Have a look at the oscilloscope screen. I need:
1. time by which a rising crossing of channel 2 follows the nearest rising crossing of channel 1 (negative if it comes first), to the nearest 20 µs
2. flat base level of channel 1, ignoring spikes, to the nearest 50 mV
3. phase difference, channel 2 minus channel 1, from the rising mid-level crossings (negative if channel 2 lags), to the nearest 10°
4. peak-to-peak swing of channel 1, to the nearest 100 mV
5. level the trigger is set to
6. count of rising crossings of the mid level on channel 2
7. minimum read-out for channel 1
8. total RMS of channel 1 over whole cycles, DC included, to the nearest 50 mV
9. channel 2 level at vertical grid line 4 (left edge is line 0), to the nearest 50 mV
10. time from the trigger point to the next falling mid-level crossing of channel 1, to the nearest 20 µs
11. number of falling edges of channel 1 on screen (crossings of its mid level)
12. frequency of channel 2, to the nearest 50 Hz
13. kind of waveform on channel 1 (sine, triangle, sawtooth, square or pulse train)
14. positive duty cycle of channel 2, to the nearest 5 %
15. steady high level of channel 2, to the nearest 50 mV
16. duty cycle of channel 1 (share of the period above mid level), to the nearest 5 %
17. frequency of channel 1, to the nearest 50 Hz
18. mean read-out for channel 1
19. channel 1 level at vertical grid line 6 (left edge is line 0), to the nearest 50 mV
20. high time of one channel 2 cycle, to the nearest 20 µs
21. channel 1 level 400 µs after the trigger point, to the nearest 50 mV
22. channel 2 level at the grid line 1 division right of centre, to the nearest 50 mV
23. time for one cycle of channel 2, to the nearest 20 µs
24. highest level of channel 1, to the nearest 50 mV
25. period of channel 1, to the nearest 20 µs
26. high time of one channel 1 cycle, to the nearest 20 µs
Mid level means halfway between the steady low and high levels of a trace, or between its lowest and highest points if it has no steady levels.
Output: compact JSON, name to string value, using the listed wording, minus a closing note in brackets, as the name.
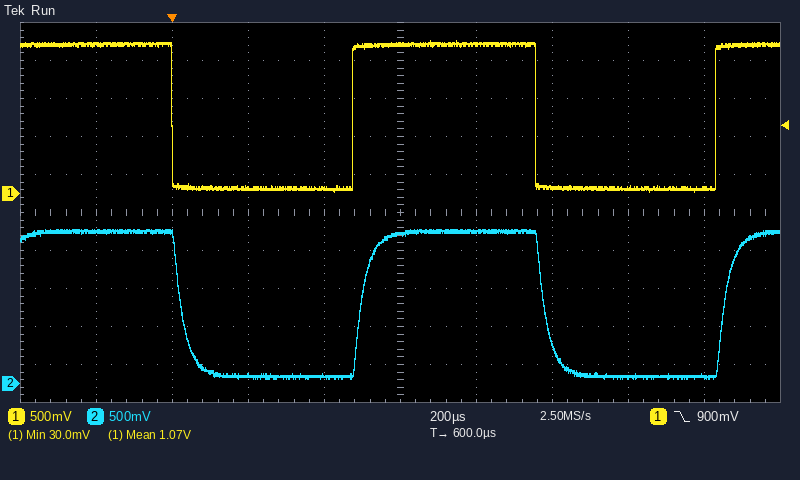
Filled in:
{"time by which a rising crossing of channel 2 follows the nearest rising crossing of channel 1 (negative if it comes first), to the nearest 20 µs": "+20 µs", "flat base level of channel 1, ignoring spikes, to the nearest 50 mV": "50 mV", "phase difference, channel 2 minus channel 1, from the rising mid-level crossings (negative if channel 2 lags), to the nearest 10°": "-10°", "peak-to-peak swing of channel 1, to the nearest 100 mV": "2.00 V", "level the trigger is set to": "900 mV", "count of rising crossings of the mid level on channel 2": "2", "minimum read-out for channel 1": "30.0 mV", "total RMS of channel 1 over whole cycles, DC included, to the nearest 50 mV": "1.40 V", "channel 2 level at vertical grid line 4 (left edge is line 0), to the nearest 50 mV": "100 mV", "time from the trigger point to the next falling mid-level crossing of channel 1, to the nearest 20 µs": "960 µs", "number of falling edges of channel 1 on screen": "2", "frequency of channel 2, to the nearest 50 Hz": "1.05 kHz", "kind of waveform on channel 1": "square", "positive duty cycle of channel 2, to the nearest 5 %": "50 %", "steady high level of channel 2, to the nearest 50 mV": "2.00 V", "duty cycle of channel 1 (share of the period above mid level), to the nearest 5 %": "50 %", "frequency of channel 1, to the nearest 50 Hz": "1.05 kHz", "mean read-out for channel 1": "1.07 V", "channel 1 level at vertical grid line 6 (left edge is line 0), to the nearest 50 mV": "1.95 V", "high time of one channel 2 cycle, to the nearest 20 µs": "480 µs", "channel 1 level 400 µs after the trigger point, to the nearest 50 mV": "50 mV", "channel 2 level at the grid line 1 division right of centre, to the nearest 50 mV": "2.00 V", "time for one cycle of channel 2, to the nearest 20 µs": "960 µs", "highest level of channel 1, to the nearest 50 mV": "2.00 V", "period of channel 1, to the nearest 20 µs": "960 µs", "high time of one channel 1 cycle, to the nearest 20 µs": "480 µs"}
